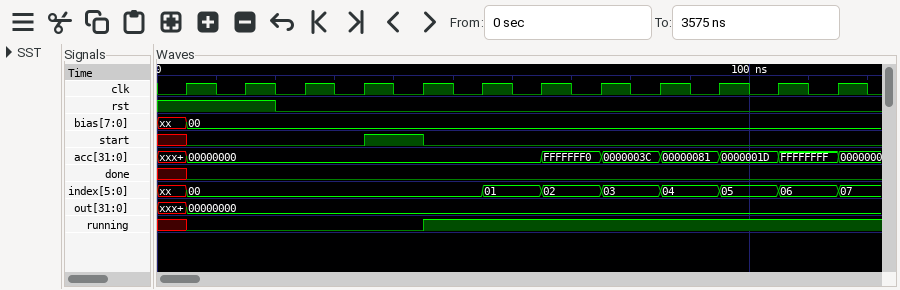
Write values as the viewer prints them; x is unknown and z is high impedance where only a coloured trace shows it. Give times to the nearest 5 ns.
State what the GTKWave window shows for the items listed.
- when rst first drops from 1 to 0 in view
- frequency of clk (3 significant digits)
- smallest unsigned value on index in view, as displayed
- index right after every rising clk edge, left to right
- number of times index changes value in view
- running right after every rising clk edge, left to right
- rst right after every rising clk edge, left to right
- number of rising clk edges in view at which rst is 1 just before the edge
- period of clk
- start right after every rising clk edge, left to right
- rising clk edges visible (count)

20 ns
100 MHz
00
00, 00, 00, 00, 00, 01, 02, 03, 04, 05, 06, 07
8
0 0 0 0 1 1 1 1 1 1 1 1
1 1 0 0 0 0 0 0 0 0 0 0
2
10 ns
0 0 0 1 0 0 0 0 0 0 0 0
12
